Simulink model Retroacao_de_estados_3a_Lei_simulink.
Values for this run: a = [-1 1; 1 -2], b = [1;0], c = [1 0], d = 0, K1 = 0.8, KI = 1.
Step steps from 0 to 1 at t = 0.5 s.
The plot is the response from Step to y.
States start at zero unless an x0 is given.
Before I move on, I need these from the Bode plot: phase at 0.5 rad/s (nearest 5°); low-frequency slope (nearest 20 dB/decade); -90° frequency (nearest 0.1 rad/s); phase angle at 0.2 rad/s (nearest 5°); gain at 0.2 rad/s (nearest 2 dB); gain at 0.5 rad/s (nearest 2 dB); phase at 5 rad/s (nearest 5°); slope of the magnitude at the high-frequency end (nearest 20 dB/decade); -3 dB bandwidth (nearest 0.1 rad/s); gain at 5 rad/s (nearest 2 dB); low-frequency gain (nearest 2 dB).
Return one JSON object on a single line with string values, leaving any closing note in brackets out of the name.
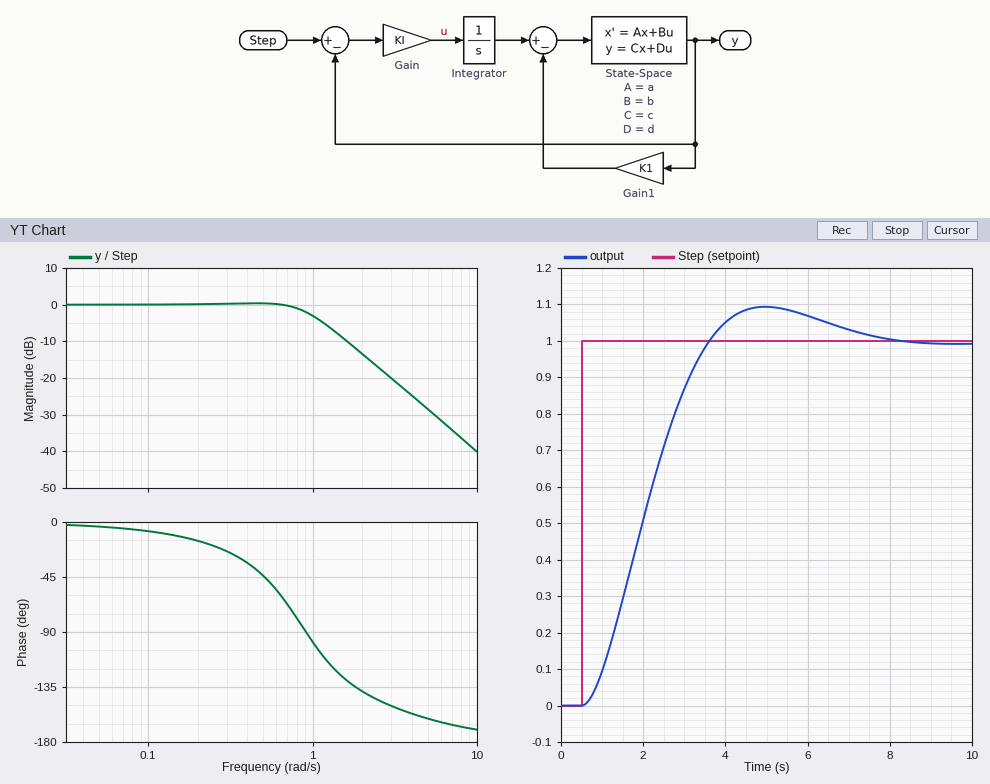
{"phase at 0.5 rad/s": "-45°", "low-frequency slope": "0 dB/decade", "-90° frequency": "0.9 rad/s", "phase angle at 0.2 rad/s": "-15°", "gain at 0.2 rad/s": "0 dB", "gain at 0.5 rad/s": "0 dB", "phase at 5 rad/s": "-160°", "slope of the magnitude at the high-frequency end": "-40 dB/decade", "-3 dB bandwidth": "1.0 rad/s", "gain at 5 rad/s": "-28 dB", "low-frequency gain": "0 dB"}
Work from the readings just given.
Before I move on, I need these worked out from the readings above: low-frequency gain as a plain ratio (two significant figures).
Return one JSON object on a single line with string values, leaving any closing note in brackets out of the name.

{"low-frequency gain as a plain ratio": "1.0"}
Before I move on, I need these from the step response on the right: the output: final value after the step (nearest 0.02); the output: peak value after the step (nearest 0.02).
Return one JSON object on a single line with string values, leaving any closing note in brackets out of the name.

{"the output: final value after the step": "1.00", "the output: peak value after the step": "1.10"}
